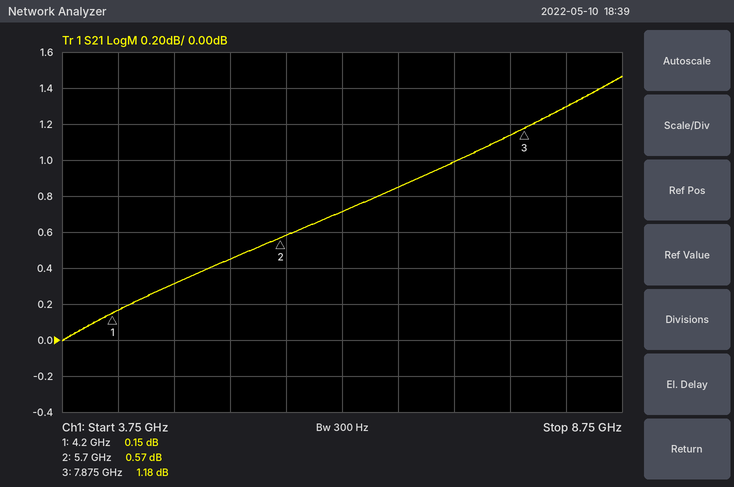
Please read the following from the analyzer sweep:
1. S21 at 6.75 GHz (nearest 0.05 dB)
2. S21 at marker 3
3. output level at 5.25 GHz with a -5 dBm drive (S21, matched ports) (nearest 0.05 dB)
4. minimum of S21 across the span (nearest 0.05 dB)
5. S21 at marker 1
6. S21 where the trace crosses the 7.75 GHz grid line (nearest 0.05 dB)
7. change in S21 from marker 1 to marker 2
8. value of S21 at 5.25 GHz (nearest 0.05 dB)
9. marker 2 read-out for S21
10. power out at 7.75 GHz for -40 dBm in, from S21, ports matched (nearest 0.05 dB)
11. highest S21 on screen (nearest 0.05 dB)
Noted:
0.85 dB
1.18 dB
-4.55 dBm
0.00 dB
0.15 dB
1.15 dB
0.42 dB
0.45 dB
0.57 dB
-38.85 dBm
1.45 dB
